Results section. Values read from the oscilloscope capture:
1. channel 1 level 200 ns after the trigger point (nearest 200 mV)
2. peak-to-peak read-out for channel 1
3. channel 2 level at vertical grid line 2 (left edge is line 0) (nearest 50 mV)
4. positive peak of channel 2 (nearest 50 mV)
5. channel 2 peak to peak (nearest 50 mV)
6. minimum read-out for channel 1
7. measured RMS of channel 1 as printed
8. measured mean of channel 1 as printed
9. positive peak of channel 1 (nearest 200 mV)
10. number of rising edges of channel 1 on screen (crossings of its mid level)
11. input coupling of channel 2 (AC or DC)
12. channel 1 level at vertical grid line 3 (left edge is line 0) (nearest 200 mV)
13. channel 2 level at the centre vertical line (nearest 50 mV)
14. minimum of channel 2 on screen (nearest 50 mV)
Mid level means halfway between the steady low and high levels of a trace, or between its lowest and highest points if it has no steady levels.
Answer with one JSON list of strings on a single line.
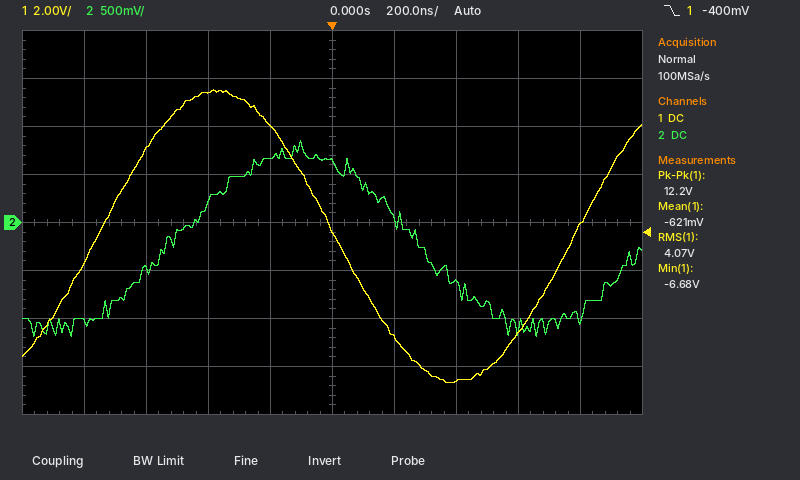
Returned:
["-4.8 V", "12.2 V", "-500 mV", "850 mV", "2.05 V", "-6.68 V", "4.07 V", "-621 mV", "5.6 V", "2", "DC", "5.4 V", "650 mV", "-1.20 V"]
